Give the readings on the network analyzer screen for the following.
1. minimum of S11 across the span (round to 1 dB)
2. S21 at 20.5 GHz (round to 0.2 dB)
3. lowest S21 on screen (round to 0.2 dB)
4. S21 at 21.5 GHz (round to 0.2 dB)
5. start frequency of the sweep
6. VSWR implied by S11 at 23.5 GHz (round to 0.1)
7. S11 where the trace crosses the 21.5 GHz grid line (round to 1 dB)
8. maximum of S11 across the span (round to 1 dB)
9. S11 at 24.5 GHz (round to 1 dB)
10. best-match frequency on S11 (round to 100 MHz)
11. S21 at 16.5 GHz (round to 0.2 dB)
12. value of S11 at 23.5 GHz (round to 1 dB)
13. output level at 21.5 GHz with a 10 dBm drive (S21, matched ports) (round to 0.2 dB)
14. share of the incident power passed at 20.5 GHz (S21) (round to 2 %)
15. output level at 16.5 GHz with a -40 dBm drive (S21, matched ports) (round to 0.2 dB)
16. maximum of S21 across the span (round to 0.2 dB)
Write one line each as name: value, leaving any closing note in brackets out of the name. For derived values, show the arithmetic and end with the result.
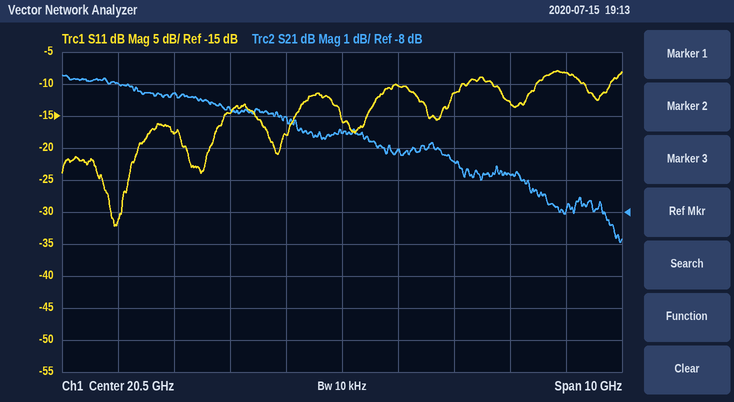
minimum of S11 across the span: -32 dB
S21 at 20.5 GHz: -5.6 dB
lowest S21 on screen: -9.0 dB
S21 at 21.5 GHz: -6.0 dB
start frequency of the sweep: 15.5 GHz
VSWR implied by S11 at 23.5 GHz: |Γ| = 10^(-13/20) = 0.2239; VSWR = (1 + 0.2239)/(1 − 0.2239) ≈ 1.6
S11 where the trace crosses the 21.5 GHz grid line: -10 dB
maximum of S11 across the span: -8 dB
S11 at 24.5 GHz: -8 dB
best-match frequency on S11: 16.4 GHz
S21 at 16.5 GHz: -4.0 dB
value of S11 at 23.5 GHz: -13 dB
output level at 21.5 GHz with a 10 dBm drive (S21, matched ports): 10 dBm + (-6.0 dB) = 4.0 dBm
share of the incident power passed at 20.5 GHz (S21): 10^(-5.6/10) ≈ 28 %
output level at 16.5 GHz with a -40 dBm drive (S21, matched ports): -40 dBm + (-4.0 dB) = -44.0 dBm
maximum of S21 across the span: -3.8 dB
